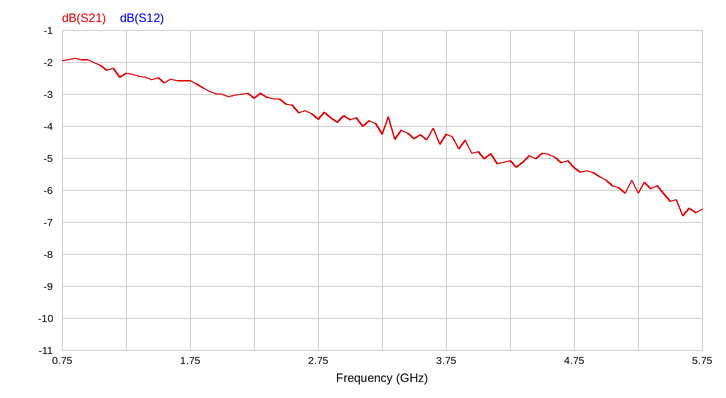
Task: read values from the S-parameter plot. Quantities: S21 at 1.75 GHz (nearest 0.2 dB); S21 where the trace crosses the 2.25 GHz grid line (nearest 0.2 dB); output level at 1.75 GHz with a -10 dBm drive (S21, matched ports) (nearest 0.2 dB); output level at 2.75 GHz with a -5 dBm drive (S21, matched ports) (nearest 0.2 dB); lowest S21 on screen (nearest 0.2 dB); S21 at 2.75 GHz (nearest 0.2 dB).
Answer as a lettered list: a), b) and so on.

a) -2.6 dB
b) -3.2 dB
c) -12.6 dBm
d) -8.8 dBm
e) -6.8 dB
f) -3.8 dB
